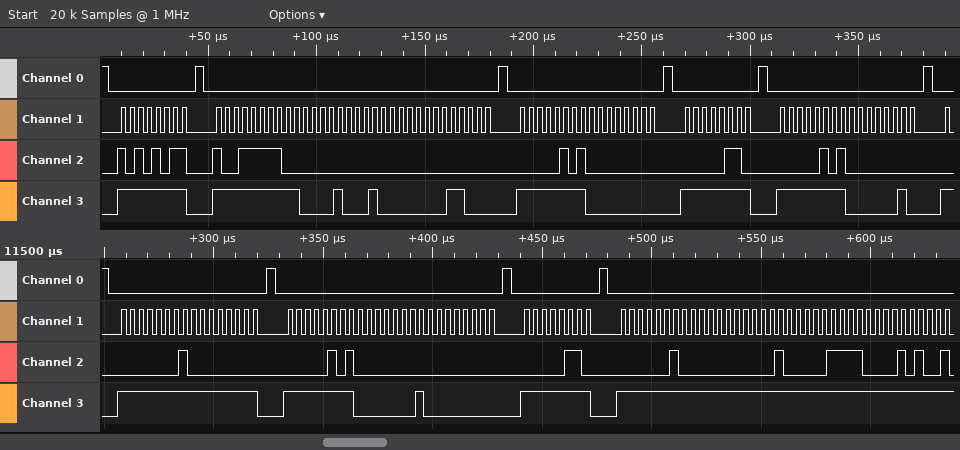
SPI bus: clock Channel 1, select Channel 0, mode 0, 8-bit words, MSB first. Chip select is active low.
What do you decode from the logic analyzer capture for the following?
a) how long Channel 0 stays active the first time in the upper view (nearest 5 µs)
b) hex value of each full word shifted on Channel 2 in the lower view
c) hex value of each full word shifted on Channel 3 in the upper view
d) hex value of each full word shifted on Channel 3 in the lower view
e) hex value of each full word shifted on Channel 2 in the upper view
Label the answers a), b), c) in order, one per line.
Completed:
a) 40 µs
b) 01, 00, 05, 00, 00, 06, 02, 00, 20, F0
c) FF, FF, C2, 20, 18, FF, 00, FF, FF, 02
d) FF, FF, FF, 01, 00, FF, FF, FF, FF, FF
e) AB, 9F, 00, 00, 00, 05, 00, 06, 05, 00
